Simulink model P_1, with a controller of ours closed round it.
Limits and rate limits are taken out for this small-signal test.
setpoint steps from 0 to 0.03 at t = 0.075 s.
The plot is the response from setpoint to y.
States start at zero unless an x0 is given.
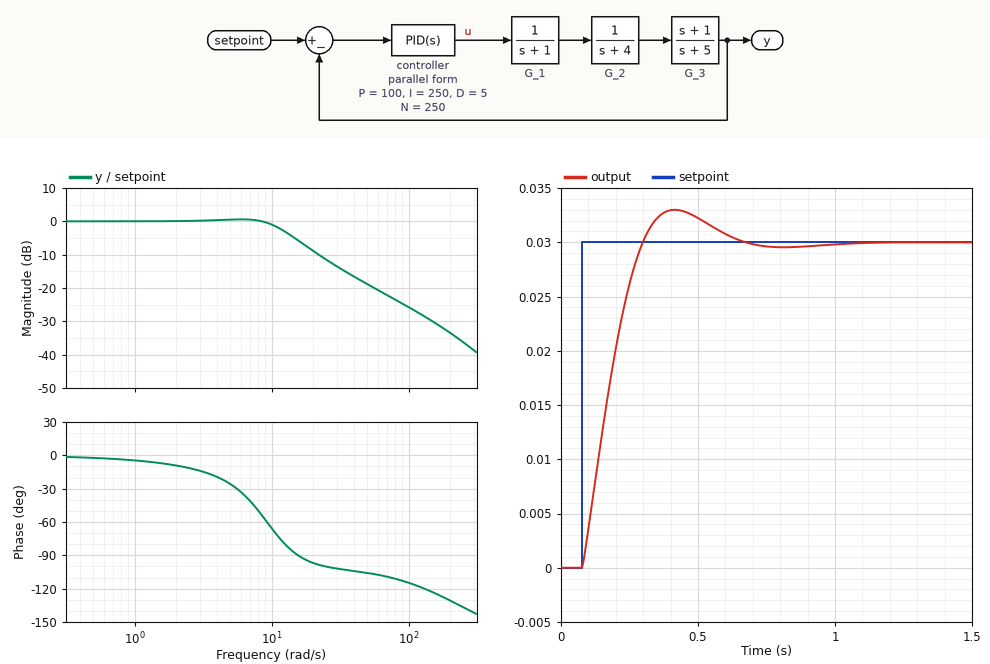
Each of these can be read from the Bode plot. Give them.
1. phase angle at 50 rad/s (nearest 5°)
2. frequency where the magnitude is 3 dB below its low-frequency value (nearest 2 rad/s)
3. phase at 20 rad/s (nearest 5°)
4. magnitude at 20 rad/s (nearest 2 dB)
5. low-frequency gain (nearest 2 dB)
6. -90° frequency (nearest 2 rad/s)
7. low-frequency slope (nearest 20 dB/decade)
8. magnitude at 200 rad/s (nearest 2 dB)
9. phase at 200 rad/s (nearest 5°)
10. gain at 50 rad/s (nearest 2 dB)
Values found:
-105°
12 rad/s
-95°
-8 dB
0 dB
16 rad/s
0 dB/decade
-34 dB
-130°
-18 dB
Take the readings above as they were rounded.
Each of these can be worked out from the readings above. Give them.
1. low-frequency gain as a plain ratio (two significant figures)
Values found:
1.0
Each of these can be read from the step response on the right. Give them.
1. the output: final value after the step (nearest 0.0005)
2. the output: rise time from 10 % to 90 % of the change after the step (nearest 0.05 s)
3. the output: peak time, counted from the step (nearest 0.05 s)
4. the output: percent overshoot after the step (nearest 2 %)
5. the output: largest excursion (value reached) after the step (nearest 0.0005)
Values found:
0.0300
0.15 s
0.35 s
10 %
0.0330
